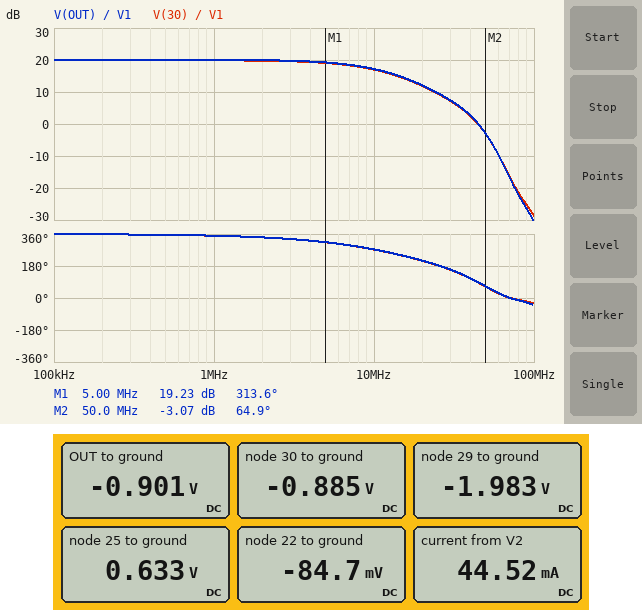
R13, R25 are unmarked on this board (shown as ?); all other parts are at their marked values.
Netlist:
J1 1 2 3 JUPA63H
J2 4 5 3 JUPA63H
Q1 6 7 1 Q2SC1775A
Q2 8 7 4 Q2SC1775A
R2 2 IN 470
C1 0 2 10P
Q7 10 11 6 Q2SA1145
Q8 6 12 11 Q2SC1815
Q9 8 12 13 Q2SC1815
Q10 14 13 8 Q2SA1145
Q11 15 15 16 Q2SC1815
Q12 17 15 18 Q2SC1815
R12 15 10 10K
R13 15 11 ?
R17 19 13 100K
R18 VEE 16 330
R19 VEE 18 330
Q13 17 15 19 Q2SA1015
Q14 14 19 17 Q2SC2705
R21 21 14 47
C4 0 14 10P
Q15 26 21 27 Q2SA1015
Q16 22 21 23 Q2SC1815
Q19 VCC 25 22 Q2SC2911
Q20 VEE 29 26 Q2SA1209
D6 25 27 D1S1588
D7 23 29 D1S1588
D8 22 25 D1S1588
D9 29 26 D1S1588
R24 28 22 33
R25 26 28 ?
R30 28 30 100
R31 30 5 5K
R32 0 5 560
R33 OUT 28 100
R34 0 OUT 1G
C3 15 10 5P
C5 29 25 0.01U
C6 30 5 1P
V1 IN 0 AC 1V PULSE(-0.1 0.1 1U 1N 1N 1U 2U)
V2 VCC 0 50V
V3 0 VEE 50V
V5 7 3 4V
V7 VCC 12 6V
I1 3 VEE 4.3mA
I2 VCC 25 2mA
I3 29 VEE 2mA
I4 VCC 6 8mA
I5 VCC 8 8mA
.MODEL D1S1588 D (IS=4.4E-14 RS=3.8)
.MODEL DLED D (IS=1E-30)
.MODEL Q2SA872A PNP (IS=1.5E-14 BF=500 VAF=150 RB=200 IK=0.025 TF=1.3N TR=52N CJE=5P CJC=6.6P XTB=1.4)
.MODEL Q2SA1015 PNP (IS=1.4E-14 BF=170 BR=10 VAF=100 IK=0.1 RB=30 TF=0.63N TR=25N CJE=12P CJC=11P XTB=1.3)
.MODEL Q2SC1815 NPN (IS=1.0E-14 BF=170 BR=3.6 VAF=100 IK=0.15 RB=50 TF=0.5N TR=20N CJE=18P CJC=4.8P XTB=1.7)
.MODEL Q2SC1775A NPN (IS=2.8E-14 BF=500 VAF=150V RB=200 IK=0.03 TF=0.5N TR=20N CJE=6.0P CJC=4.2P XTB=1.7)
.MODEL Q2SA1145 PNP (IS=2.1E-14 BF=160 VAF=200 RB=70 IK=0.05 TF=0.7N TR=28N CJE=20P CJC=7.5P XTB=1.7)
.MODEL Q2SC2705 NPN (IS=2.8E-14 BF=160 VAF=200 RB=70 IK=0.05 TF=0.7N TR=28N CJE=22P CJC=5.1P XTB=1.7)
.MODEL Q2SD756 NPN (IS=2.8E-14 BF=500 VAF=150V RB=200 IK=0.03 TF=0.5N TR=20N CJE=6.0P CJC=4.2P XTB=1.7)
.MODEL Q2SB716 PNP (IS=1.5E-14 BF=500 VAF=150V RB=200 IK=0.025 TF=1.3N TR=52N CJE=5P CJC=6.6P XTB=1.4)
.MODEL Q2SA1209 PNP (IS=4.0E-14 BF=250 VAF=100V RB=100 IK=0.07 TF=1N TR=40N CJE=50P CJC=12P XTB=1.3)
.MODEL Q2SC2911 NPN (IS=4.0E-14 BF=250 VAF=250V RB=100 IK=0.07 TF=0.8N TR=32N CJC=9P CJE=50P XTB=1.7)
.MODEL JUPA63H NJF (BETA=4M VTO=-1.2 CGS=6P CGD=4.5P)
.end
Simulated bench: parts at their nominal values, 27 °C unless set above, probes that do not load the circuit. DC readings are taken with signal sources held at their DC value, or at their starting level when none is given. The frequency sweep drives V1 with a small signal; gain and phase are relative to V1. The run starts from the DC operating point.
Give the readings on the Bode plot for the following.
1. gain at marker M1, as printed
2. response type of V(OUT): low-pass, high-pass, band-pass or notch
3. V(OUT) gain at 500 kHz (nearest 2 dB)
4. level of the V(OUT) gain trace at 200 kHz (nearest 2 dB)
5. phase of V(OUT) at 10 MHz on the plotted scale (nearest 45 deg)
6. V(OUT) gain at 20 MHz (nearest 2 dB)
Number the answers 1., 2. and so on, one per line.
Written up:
1. 19.23 dB
2. low-pass
3. 20 dB
4. 20 dB
5. 270 deg
6. 12 dB
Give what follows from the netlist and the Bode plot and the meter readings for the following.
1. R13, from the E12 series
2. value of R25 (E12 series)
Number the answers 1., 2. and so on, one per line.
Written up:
1. 220 kΩ
2. 15 Ω
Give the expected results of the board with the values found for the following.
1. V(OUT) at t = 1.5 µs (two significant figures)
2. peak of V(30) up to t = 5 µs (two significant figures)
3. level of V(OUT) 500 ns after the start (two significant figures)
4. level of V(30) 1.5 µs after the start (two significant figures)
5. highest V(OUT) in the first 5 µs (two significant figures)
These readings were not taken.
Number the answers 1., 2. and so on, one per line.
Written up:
1. 1.1 V
2. 1.1 V
3. -900 mV
4. 1.1 V
5. 1.1 V
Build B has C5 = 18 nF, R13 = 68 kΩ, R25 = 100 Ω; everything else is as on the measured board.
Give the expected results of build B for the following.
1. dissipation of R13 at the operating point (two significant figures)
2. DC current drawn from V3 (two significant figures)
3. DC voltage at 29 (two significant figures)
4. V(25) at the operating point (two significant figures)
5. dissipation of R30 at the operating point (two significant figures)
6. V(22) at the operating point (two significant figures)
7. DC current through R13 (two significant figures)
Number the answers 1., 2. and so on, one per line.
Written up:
1. 120 mW
2. 29 mA
3. -2.5 V
4. 83 mV
5. 2.6 µW
6. -600 mV
7. 1.3 mA
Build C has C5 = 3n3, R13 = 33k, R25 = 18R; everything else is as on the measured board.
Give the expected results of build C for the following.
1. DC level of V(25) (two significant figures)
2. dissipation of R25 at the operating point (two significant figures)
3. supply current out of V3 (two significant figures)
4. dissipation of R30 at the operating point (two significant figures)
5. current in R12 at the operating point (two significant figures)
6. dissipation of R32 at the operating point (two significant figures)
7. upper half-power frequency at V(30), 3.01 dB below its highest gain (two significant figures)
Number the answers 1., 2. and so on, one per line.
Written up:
1. 560 mV
2. 10 mW
3. 43 mA
4. 2.7 µW
5. 3.1 mA
6. 15 µW
7. 9.8 MHz
